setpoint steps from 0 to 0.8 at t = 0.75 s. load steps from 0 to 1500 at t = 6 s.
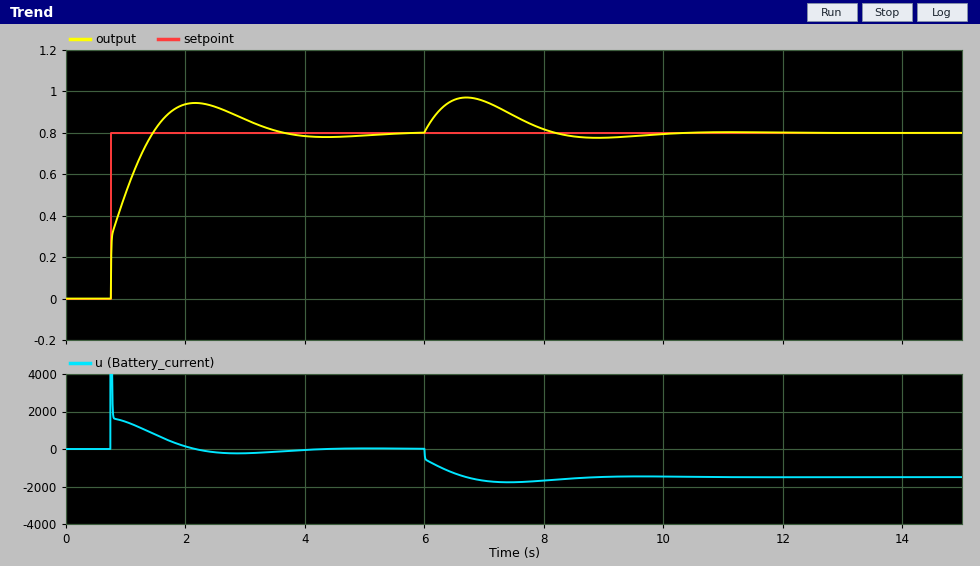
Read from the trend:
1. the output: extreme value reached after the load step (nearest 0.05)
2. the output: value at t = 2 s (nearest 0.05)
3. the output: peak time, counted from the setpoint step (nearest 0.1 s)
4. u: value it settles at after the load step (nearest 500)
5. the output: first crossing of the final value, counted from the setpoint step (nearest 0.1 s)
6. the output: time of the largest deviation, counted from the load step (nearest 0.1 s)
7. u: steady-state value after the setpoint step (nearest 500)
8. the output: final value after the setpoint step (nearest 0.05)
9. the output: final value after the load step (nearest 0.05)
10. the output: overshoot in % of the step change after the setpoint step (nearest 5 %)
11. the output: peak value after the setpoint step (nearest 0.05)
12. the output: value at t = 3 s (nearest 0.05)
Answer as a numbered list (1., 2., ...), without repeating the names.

1. 0.95
2. 0.95
3. 1.4 s
4. -1500
5. 0.7 s
6. 0.7 s
7. 0
8. 0.80
9. 0.80
10. 20 %
11. 0.95
12. 0.85
